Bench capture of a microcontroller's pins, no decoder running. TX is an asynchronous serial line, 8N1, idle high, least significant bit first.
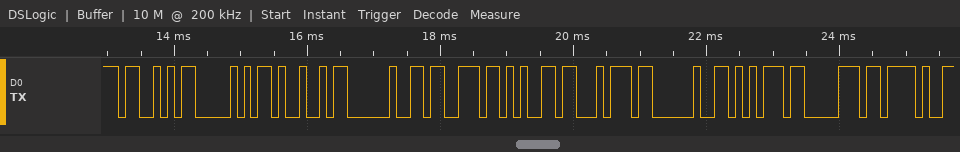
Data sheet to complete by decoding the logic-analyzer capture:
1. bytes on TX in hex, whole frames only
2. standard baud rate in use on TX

0x53 0x50 0x49 0x20 0x73 0x65 0x74 0x20 0x75 0x70 0x2F
9600 baud
